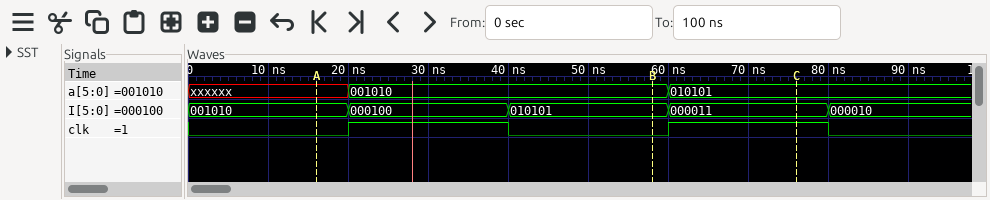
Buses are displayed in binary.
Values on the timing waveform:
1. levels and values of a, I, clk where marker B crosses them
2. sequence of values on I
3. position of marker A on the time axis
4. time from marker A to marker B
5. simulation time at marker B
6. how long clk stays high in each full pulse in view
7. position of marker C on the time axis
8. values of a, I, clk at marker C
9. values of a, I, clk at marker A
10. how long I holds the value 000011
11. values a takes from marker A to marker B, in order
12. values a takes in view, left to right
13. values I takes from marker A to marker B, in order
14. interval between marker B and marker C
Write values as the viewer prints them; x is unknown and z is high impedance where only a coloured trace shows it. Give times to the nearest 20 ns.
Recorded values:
a=001010, I=010101, clk=0
001010, 000100, 010101, 000011, 000010
20 ns
40 ns
60 ns
20 ns, 20 ns
80 ns
a=010101, I=000011, clk=1
a=xxxxxx, I=001010, clk=0
20 ns
xxxxxx, 001010
xxxxxx, 001010, 010101
001010, 000100, 010101
20 ns
